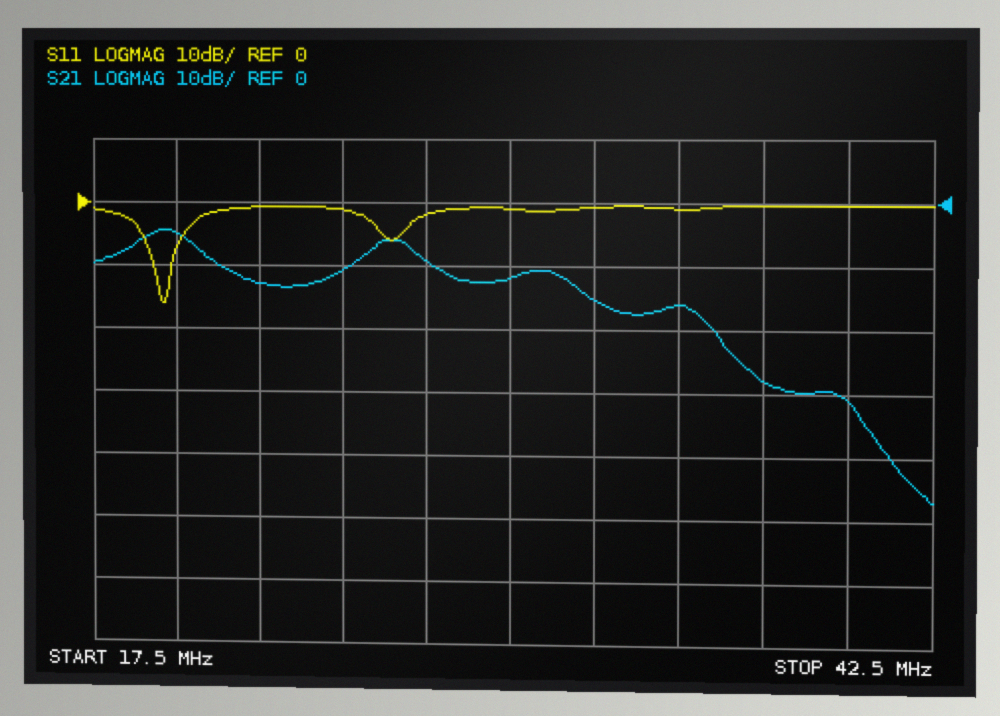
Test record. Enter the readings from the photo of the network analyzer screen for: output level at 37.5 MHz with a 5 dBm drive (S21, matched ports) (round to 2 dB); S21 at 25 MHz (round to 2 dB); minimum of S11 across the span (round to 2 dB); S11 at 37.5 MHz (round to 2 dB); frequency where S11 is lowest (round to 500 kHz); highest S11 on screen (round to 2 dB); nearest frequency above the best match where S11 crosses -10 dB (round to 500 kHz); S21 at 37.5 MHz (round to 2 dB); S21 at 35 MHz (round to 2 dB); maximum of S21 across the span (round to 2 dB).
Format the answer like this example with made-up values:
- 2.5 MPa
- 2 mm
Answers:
- -22 dBm
- -10 dB
- -16 dB
- 0 dB
- 19.5 MHz
- 0 dB
- 20.0 MHz
- -28 dB
- -16 dB
- -4 dB
